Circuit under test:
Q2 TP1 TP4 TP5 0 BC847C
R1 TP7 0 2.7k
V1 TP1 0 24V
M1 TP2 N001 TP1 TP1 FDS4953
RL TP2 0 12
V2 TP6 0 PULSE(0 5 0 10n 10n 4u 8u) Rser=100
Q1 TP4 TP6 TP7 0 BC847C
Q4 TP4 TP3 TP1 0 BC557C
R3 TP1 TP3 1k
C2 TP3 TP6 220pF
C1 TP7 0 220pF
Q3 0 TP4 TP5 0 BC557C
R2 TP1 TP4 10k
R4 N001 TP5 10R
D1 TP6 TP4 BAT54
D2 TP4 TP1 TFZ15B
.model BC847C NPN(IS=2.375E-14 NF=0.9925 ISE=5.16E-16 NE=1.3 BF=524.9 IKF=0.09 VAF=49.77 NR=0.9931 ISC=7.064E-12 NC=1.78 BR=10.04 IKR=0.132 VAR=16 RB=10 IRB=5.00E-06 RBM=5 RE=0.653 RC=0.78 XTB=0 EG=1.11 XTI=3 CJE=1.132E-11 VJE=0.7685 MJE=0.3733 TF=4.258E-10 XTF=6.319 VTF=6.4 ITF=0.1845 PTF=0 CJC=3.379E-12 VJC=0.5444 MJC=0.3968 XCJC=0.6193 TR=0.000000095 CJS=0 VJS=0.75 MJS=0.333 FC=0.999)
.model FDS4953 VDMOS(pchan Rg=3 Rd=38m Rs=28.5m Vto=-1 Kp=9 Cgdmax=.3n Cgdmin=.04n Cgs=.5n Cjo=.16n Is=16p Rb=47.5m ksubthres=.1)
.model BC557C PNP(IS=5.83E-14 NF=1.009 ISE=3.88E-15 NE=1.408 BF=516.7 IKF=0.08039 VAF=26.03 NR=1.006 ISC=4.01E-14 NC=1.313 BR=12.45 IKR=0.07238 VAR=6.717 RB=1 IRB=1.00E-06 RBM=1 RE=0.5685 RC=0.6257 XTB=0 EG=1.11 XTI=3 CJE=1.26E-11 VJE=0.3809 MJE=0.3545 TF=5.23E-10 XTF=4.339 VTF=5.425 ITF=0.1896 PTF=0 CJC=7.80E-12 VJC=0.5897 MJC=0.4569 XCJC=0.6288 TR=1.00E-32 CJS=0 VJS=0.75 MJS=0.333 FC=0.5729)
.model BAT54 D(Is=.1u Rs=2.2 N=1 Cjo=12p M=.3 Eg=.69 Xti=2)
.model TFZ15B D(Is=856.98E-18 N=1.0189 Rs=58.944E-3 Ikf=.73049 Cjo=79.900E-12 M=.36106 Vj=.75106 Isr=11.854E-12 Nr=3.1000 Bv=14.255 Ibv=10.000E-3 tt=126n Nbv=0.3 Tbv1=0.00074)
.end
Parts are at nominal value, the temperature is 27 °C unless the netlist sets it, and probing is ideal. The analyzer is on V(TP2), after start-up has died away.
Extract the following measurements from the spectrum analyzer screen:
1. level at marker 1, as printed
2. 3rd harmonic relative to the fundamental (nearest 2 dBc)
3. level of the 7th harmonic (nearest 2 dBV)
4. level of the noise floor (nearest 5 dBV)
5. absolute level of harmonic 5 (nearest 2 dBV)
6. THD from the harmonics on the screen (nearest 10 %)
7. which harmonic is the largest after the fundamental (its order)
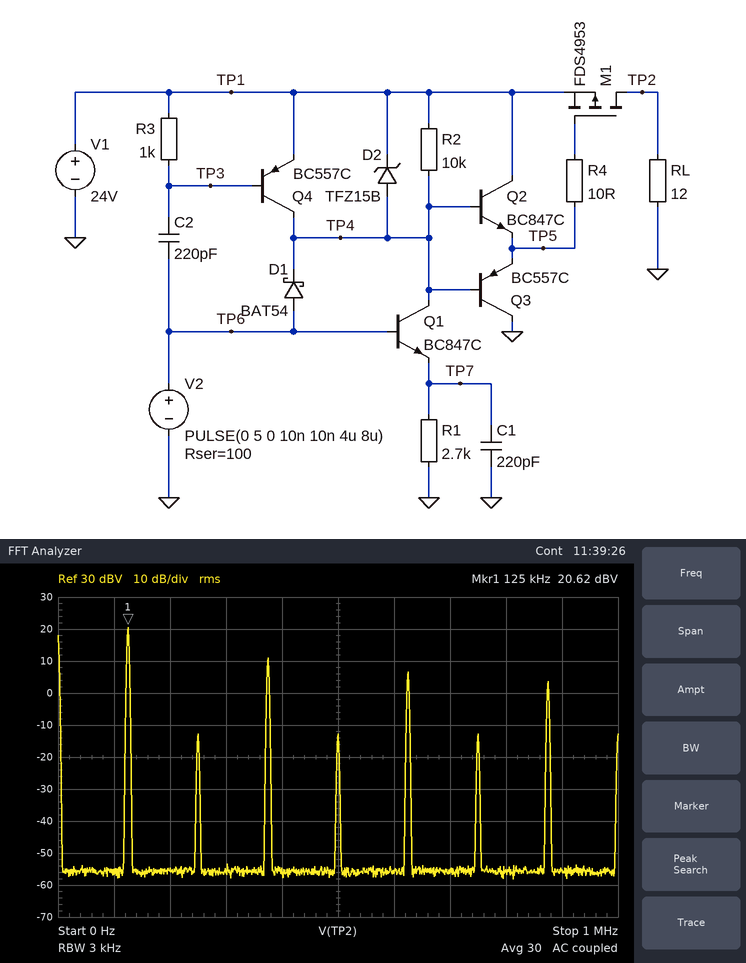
20.62 dBV
-10 dBc
4 dBV
-55 dBV
6 dBV
40 %
3
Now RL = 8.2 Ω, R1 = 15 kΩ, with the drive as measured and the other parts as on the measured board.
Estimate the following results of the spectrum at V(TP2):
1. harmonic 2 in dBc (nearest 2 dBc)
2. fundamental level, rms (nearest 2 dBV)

-38 dBc
20 dBV
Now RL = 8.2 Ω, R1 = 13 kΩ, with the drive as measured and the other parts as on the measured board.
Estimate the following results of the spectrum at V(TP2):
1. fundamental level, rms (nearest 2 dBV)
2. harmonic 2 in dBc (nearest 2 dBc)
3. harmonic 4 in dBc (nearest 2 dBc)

20 dBV
-38 dBc
-38 dBc
